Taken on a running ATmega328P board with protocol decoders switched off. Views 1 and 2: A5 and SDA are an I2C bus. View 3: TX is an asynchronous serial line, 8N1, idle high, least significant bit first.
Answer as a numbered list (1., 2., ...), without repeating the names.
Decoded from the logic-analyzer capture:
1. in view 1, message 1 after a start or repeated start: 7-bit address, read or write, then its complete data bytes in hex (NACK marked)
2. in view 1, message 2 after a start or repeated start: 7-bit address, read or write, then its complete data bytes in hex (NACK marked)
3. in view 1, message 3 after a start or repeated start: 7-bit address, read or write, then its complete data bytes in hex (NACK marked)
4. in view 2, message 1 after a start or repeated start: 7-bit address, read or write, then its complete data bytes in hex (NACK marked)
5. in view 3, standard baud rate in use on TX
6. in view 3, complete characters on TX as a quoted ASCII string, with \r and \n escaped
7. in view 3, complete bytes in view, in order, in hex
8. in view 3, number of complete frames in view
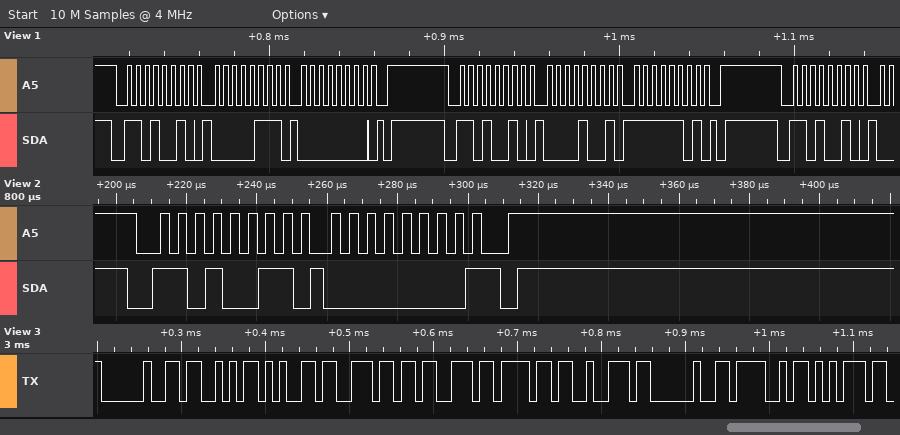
1. 0x69 write: 07 00
2. 0x69 write: 09 FD
3. 0x69 write
4. 0x69 read: 00 NACK
5. 115200 baud
6. " Sensor Ou"
7. 20 53 65 6E 73 6F 72 20 4F 75
8. 10
